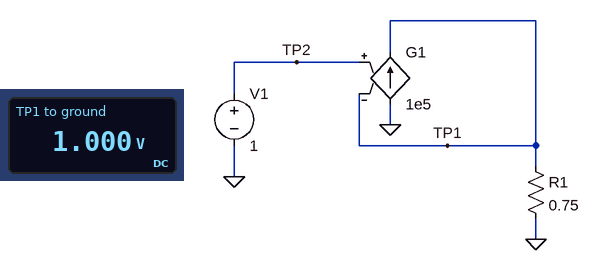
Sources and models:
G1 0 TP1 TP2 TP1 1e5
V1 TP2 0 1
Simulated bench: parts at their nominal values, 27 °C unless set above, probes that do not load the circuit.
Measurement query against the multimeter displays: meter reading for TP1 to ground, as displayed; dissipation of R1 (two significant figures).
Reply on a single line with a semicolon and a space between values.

1.000 V; 1.3 W
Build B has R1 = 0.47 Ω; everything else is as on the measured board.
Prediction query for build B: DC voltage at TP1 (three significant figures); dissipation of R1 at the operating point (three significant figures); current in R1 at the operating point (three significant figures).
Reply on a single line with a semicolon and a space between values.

1.00 V; 2.13 W; 2.13 A
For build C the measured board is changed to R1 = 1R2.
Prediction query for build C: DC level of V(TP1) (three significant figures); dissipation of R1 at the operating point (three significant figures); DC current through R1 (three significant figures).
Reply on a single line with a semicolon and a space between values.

1.00 V; 833 mW; 833 mA
